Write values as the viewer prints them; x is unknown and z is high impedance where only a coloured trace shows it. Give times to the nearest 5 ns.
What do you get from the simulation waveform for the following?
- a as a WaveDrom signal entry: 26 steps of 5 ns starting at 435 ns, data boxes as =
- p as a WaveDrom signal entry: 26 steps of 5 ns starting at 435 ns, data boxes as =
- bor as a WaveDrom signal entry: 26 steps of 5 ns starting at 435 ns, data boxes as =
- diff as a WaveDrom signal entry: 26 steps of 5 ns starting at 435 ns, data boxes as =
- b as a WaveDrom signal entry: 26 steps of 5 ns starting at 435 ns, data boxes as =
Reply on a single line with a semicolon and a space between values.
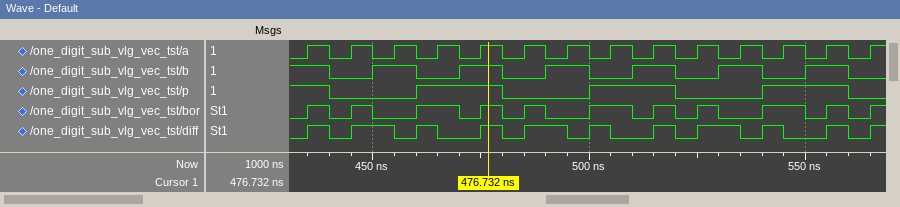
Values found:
{name: 'a', wave: '10101010101010101010101010'}; {name: 'p', wave: '10...1...0...1...0...1...0'}; {name: 'bor', wave: '1010.1.01010.1.01010.1.010'}; {name: 'diff', wave: '101.010.101.010.101.010.10'}; {name: 'b', wave: '10.1.0.1.0.1.0.1.0.1.0.1.0'}
